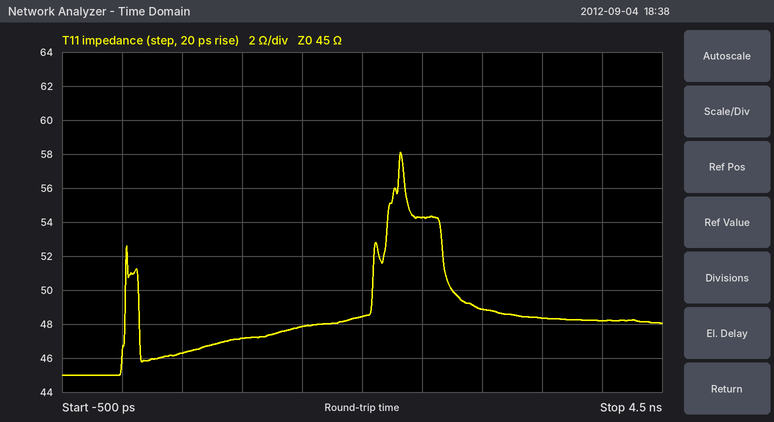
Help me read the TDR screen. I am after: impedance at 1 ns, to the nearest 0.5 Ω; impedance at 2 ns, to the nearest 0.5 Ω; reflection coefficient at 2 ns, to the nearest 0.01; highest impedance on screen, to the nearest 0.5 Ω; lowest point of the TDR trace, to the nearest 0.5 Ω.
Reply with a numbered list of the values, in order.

1. 47.0 Ω
2. 48.5 Ω
3. +0.04
4. 58.0 Ω
5. 45.0 Ω
